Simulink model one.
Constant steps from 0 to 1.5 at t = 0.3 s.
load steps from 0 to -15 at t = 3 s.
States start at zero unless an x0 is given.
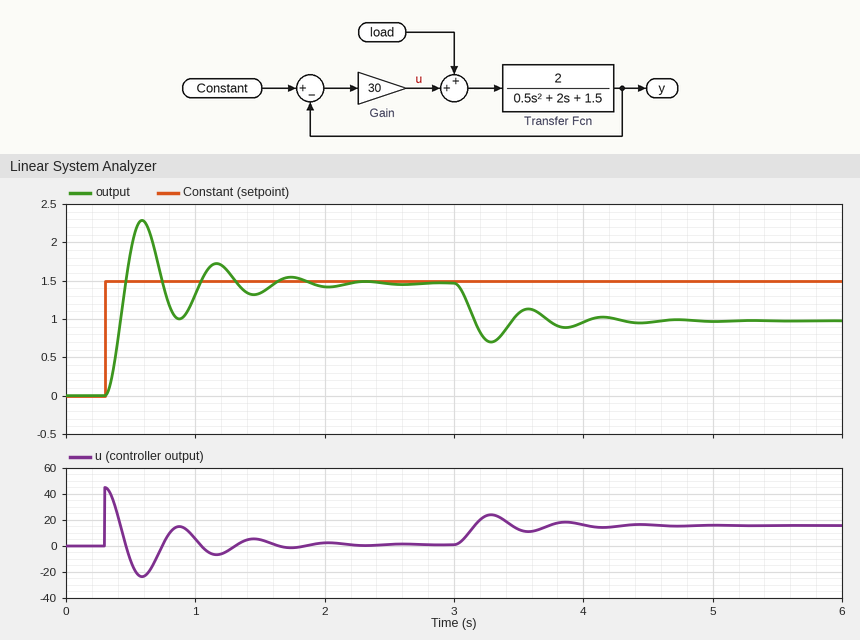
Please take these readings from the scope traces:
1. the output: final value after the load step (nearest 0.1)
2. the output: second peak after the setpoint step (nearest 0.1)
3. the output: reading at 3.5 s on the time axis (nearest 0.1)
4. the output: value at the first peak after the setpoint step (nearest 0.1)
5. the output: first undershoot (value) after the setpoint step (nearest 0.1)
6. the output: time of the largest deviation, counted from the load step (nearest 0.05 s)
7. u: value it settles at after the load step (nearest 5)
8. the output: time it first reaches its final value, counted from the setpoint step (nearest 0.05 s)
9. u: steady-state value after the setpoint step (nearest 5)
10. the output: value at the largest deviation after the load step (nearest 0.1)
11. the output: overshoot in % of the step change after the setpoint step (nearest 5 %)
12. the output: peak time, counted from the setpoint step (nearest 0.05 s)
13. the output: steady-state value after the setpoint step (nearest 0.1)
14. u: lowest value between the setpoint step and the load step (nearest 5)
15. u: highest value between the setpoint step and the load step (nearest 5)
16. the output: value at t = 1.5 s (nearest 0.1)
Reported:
1.0
1.7
1.1
2.3
1.0
0.30 s
15
0.15 s
0
0.7
55 %
0.30 s
1.5
-25
45
1.3
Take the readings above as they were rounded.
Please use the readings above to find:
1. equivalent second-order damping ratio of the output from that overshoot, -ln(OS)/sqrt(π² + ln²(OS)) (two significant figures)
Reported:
0.19
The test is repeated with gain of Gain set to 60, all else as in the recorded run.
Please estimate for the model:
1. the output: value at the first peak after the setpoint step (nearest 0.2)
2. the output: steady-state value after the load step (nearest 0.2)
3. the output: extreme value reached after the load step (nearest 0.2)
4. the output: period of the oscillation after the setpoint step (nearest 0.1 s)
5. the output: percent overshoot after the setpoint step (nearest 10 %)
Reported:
2.4
1.2
1.0
0.4 s
70 %
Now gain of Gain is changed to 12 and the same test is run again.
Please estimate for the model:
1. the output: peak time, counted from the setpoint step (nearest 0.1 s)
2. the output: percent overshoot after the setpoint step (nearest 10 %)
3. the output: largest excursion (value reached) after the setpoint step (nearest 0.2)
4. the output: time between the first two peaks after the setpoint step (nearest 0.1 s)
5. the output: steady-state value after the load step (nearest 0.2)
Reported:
0.5 s
40 %
2.0
0.9 s
0.2
